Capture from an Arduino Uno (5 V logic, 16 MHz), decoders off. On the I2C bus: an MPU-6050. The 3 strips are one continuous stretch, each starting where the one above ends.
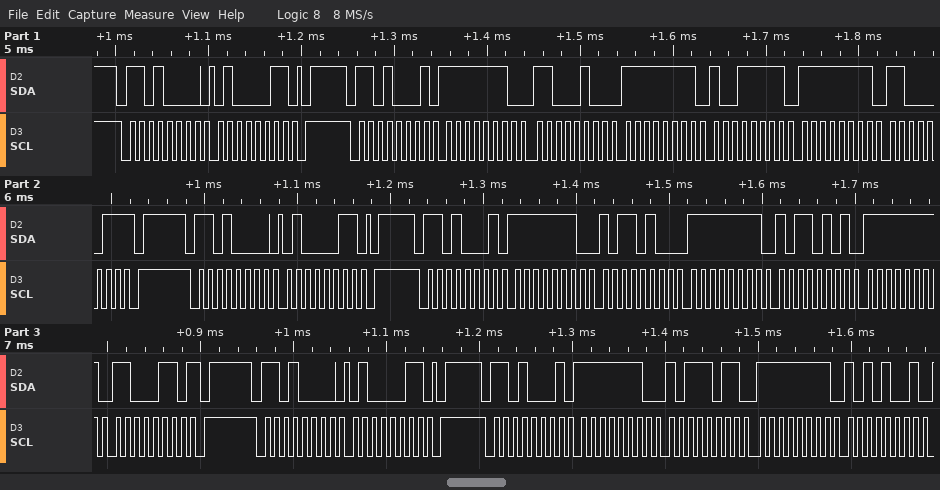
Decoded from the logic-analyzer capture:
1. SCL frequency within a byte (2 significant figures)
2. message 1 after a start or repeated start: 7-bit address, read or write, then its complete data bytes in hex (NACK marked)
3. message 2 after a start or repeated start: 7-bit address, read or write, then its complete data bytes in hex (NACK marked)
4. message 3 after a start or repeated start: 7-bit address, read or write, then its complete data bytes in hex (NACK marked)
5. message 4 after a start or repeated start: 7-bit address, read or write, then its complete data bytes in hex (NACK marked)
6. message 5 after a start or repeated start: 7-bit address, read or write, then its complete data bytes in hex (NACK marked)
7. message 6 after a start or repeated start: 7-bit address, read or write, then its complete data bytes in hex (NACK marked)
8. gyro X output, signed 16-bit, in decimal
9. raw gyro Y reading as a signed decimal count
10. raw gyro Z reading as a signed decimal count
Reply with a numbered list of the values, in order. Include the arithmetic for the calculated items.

1. 100 kHz
2. 0x68 write: 43
3. 0x68 read: FE C4 FF 9F FF C3 NACK
4. 0x68 write: 43
5. 0x68 read: FE B4 FF B5 FF C6 NACK
6. 0x68 write: 43
7. 0x68 read: FE BB FF A9
8. 0xFEC4 = -316
9. 0xFF9F = -97
10. 0xFFC3 = -61
